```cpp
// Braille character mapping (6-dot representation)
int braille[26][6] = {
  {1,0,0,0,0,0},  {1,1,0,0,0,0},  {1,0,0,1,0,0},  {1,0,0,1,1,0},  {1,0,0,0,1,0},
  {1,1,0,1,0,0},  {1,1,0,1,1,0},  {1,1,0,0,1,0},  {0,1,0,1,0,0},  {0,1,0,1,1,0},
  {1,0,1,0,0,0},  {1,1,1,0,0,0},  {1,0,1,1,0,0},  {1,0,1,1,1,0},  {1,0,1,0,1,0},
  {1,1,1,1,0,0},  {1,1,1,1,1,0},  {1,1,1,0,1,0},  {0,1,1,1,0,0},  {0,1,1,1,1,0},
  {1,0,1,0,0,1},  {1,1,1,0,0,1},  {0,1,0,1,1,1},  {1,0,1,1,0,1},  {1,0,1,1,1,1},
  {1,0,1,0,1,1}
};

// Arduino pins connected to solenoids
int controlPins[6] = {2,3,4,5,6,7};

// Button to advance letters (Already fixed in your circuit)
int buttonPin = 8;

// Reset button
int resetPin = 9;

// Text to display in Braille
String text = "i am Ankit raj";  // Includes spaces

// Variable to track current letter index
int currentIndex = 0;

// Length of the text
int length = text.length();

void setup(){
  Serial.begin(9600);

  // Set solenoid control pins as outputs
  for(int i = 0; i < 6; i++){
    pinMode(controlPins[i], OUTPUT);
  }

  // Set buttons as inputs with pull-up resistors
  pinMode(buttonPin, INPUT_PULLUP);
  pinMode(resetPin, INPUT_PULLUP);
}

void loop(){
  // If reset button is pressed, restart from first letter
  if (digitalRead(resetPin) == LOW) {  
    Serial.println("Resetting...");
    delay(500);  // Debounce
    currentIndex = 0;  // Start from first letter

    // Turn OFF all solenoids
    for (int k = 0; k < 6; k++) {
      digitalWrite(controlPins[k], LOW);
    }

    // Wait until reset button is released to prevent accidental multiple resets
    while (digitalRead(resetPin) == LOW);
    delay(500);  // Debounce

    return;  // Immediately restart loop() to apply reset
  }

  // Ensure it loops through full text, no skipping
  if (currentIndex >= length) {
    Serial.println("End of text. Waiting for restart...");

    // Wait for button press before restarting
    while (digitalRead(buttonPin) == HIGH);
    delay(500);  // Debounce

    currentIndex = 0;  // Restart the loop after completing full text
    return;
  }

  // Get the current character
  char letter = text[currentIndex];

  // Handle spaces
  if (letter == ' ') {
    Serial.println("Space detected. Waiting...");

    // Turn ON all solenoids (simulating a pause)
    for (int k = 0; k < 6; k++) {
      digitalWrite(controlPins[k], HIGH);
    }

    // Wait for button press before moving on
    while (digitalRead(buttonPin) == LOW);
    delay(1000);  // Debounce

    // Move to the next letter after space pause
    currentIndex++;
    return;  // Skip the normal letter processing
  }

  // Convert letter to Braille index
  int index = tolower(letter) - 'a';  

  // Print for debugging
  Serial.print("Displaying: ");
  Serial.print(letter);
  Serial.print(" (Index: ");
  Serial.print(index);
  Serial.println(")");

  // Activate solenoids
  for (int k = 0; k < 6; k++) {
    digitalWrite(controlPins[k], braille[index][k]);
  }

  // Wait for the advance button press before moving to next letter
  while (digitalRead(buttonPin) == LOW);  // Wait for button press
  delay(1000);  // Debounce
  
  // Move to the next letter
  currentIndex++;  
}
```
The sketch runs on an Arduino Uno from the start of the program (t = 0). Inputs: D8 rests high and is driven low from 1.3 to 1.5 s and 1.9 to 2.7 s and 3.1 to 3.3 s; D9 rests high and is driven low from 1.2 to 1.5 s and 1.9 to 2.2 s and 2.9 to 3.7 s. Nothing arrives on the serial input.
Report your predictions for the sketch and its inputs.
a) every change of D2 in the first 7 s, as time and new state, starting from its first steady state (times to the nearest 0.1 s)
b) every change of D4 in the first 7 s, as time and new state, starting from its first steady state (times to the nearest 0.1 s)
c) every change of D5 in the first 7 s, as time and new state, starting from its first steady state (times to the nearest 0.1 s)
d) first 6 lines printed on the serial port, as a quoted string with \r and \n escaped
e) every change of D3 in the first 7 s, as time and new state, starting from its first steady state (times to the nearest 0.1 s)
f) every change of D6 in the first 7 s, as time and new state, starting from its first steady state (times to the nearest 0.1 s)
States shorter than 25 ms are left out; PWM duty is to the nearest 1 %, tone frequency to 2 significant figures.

0 s low; 1 s high; 2.5 s low; 5.2 s high
0 s low; 1 s high; 2.5 s low; 5.2 s high; 6.2 s low
0 s high; 2.5 s low; 4.2 s high; 6.2 s low
"Displaying: i (Index: 8)\r\nSpace detected. Waiting...\r\nResetting...\r\nResetting...\r\nDisplaying: i (Index: 8)\r\nSpace detected. Waiting...\r\n"
0 s high; 2.5 s low; 4.2 s high; 6.2 s low
0 s low; 1 s high; 2.5 s low; 5.2 s high; 6.2 s low
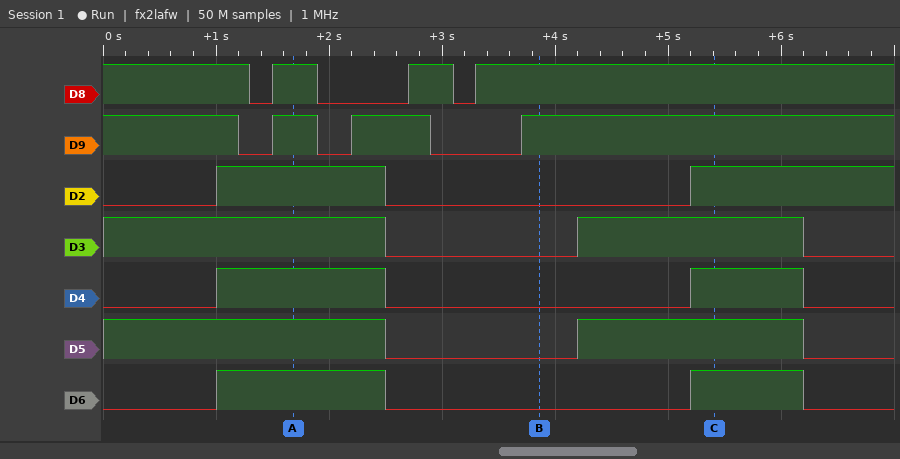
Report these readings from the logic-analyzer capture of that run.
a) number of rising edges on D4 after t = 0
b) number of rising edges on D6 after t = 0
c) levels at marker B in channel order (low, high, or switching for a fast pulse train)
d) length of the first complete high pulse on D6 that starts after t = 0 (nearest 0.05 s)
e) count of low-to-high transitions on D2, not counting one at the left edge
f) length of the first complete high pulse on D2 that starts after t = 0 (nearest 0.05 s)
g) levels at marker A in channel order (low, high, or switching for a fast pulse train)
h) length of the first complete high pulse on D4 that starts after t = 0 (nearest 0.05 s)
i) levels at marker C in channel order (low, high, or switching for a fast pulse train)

2
2
D8 high, D9 high, D2 low, D3 low, D4 low, D5 low, D6 low
1.50 s
2
1.50 s
D8 high, D9 high, D2 high, D3 high, D4 high, D5 high, D6 high
1.50 s
D8 high, D9 high, D2 high, D3 high, D4 high, D5 high, D6 high
